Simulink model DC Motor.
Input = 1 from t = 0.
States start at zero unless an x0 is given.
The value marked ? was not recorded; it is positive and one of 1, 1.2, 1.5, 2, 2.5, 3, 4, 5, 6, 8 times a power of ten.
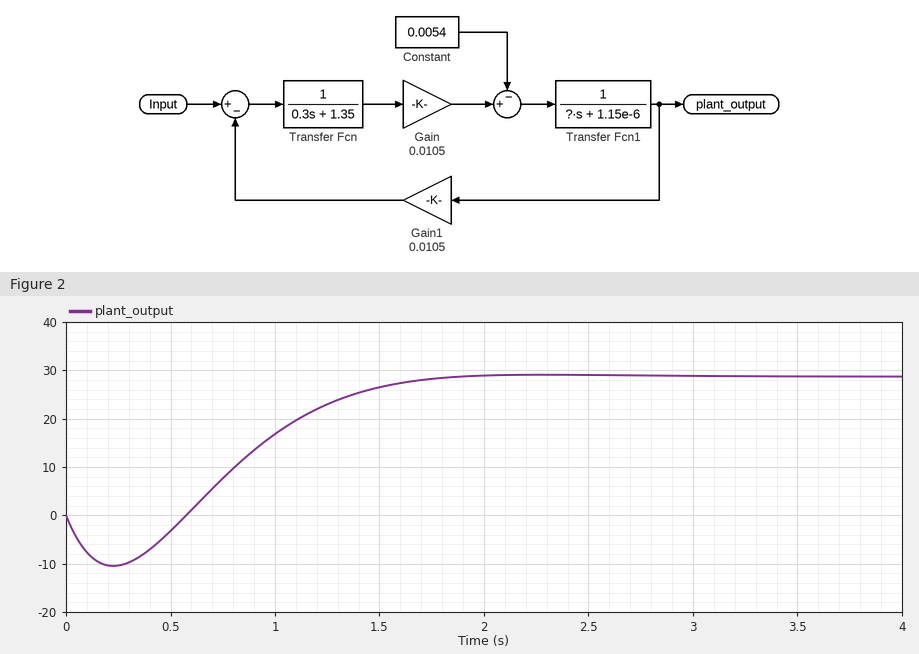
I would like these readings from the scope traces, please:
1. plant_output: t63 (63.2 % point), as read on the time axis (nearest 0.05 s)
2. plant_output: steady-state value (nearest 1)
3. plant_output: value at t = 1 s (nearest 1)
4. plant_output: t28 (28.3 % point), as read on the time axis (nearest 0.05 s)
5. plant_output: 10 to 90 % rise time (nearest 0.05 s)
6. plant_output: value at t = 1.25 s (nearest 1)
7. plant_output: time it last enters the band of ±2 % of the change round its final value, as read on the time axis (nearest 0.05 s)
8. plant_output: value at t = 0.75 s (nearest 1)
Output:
1.05 s
29
17
0.75 s
0.80 s
23
1.75 s
8
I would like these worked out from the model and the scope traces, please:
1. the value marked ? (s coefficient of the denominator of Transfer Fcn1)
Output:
5e-05
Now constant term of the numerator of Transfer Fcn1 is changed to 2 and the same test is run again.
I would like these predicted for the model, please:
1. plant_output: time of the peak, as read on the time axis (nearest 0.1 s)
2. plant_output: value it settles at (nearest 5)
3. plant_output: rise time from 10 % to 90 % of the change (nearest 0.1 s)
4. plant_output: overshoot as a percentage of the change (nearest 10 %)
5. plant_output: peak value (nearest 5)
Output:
1.2 s
30
0.3 s
20 %
35
